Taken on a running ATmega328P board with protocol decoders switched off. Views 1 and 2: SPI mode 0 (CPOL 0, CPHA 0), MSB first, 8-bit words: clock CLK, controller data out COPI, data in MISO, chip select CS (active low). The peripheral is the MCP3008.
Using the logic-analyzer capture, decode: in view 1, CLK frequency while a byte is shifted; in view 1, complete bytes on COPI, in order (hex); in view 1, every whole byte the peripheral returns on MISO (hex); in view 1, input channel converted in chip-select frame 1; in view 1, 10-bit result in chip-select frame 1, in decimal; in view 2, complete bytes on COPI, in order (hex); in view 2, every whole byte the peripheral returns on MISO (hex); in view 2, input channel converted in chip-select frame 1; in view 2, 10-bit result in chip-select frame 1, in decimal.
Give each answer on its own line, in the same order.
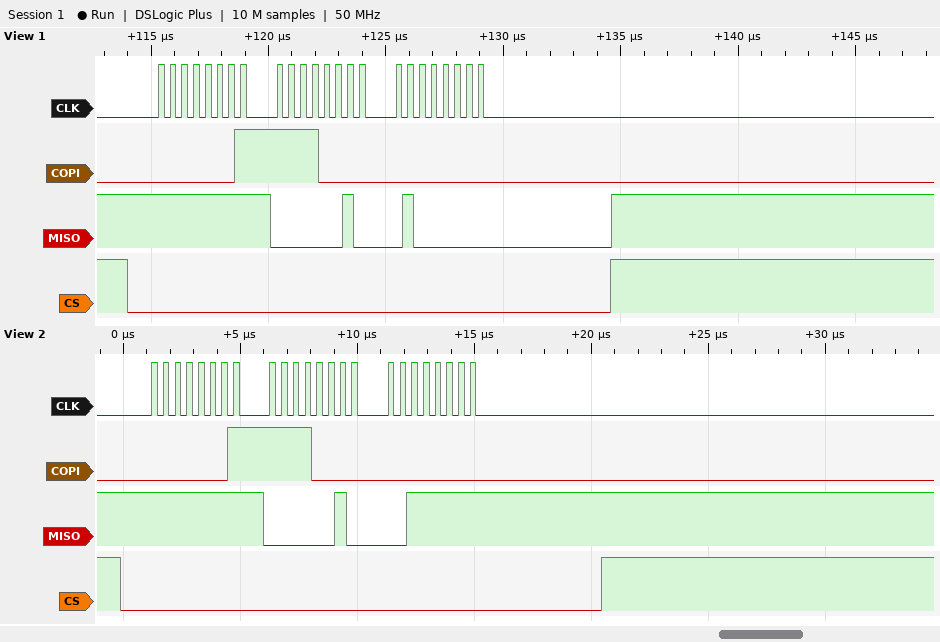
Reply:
2 MHz
01 F0 00
FF 02 40
7
576
0x01 0xF0 0x00
0xFF 0x02 0x3F
7
575
